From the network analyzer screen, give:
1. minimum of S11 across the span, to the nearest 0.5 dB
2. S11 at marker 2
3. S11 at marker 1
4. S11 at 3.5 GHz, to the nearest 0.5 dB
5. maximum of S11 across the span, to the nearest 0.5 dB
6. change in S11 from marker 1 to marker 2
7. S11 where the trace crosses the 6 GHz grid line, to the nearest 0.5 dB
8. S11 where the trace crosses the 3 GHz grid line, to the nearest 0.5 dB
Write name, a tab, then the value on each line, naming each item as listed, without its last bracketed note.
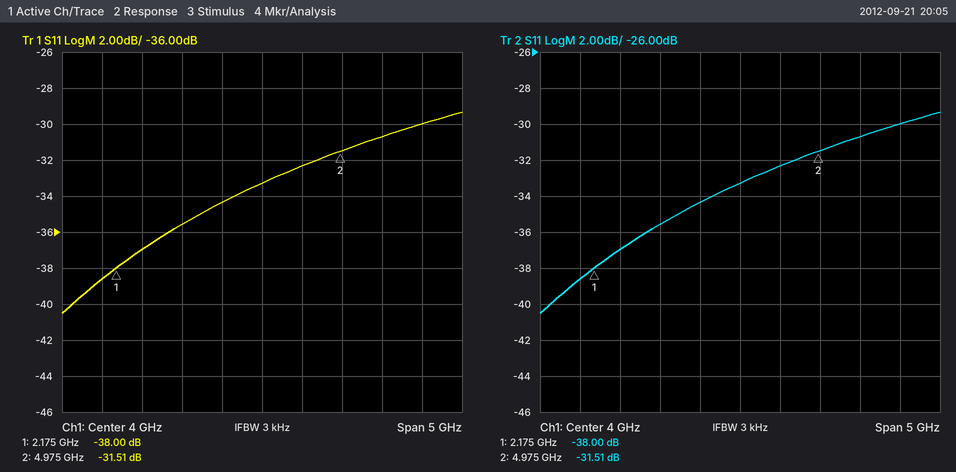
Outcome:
minimum of S11 across the span, to the nearest 0.5 dB	-40.5 dB
S11 at marker 2	-31.51 dB
S11 at marker 1	-38.00 dB
S11 at 3.5 GHz, to the nearest 0.5 dB	-34.5 dB
maximum of S11 across the span, to the nearest 0.5 dB	-29.5 dB
change in S11 from marker 1 to marker 2	6.49 dB
S11 where the trace crosses the 6 GHz grid line, to the nearest 0.5 dB	-30.0 dB
S11 where the trace crosses the 3 GHz grid line, to the nearest 0.5 dB	-35.5 dB
